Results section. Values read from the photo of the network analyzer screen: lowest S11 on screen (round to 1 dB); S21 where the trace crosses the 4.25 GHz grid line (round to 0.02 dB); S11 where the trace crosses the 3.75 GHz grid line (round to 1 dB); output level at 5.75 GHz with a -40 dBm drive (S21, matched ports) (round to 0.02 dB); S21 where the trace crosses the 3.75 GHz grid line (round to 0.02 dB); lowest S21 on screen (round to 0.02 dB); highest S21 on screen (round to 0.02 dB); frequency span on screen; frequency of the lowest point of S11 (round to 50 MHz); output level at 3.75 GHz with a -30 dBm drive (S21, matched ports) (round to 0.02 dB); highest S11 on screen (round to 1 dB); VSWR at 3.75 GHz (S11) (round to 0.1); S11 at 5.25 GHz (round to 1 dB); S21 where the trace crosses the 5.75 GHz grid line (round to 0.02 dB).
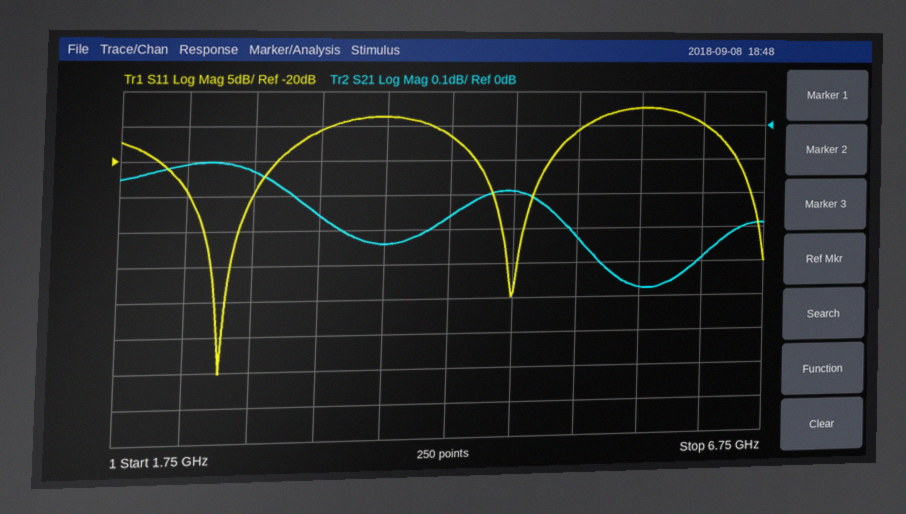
-50 dB
-0.26 dB
-14 dB
-40.48 dBm
-0.34 dB
-0.48 dB
-0.10 dB
5 GHz
2.50 GHz
-30.34 dBm
-12 dB
1.5
-16 dB
-0.48 dB
